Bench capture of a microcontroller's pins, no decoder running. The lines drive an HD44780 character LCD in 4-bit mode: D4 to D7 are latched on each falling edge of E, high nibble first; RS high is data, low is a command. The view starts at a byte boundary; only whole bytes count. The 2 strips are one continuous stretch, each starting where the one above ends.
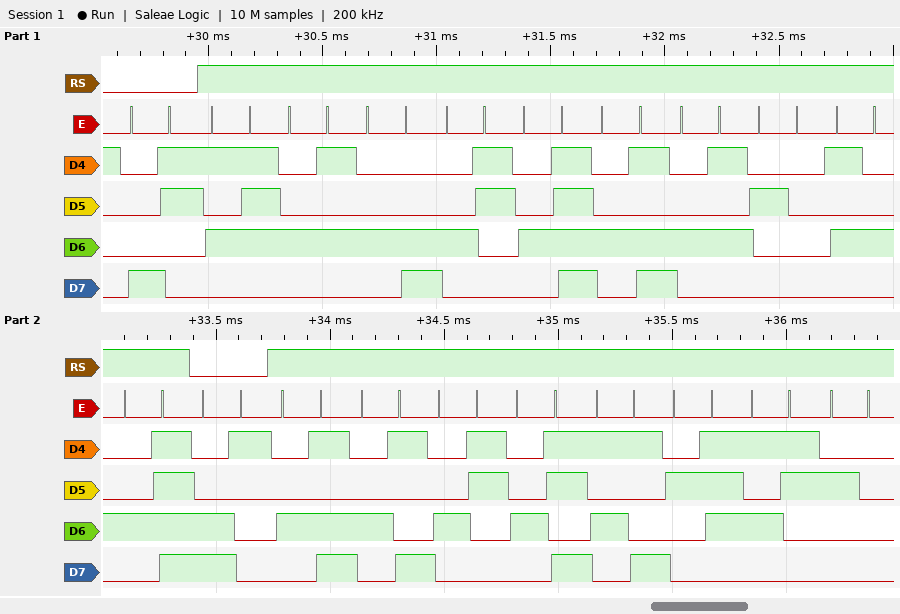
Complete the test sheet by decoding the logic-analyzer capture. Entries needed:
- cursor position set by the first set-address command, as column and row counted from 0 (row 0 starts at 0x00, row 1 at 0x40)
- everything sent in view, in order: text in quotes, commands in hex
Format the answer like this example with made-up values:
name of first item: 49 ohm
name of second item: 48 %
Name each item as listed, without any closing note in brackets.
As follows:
cursor position set by the first set-address command, as column and row counted from 0: column 3, row 0
everything sent in view, in order: text in quotes, commands in hex: 0x83 "WELCOME TO" 0xC1 "MICKY'S "
